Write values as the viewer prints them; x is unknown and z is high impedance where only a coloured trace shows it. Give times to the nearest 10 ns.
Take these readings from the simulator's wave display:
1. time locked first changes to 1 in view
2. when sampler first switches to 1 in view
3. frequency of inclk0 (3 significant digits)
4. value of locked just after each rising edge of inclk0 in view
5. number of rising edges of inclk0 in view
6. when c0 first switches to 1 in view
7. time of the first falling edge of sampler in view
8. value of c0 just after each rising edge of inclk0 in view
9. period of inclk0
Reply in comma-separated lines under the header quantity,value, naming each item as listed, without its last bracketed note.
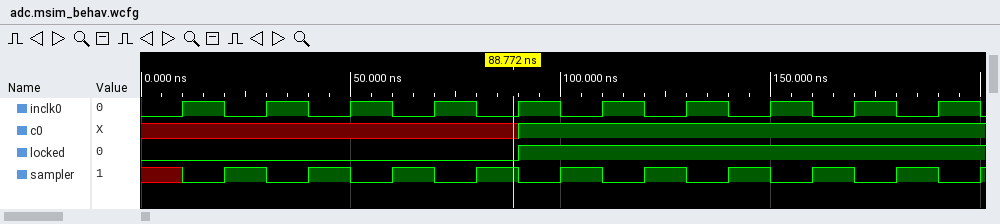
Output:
quantity,value
time locked first changes to 1 in view,90 ns
when sampler first switches to 1 in view,20 ns
frequency of inclk0,50.0 MHz
value of locked just after each rising edge of inclk0 in view,0 0 0 0 1 1 1 1 1 1
number of rising edges of inclk0 in view,10
when c0 first switches to 1 in view,90 ns
time of the first falling edge of sampler in view,30 ns
value of c0 just after each rising edge of inclk0 in view,x x x x 1 1 1 1 1 1
period of inclk0,20 ns
